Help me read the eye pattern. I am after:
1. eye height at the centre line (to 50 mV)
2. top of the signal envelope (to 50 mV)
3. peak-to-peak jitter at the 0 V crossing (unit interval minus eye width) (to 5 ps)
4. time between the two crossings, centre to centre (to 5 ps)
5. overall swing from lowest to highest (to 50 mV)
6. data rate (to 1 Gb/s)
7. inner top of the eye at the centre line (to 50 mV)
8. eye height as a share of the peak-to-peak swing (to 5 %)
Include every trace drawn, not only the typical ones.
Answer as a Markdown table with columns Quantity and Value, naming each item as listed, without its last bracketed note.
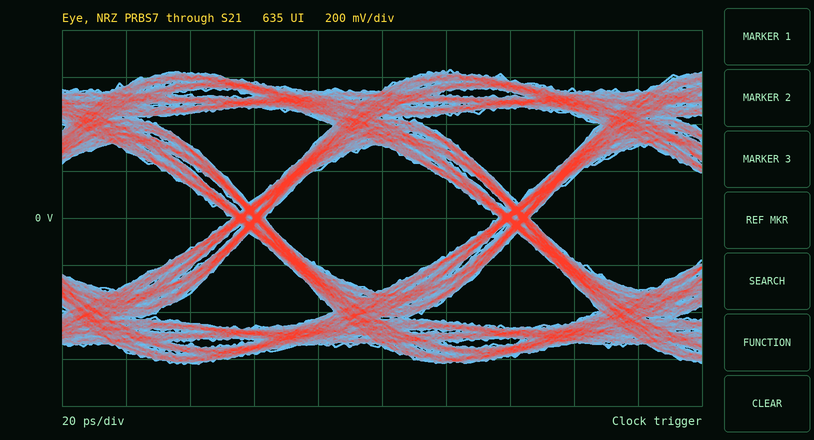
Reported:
| Quantity | Value |
|---|---|
| eye height at the centre line | 600 mV |
| top of the signal envelope | 650 mV |
| peak-to-peak jitter at the 0 V crossing (unit interval minus eye width) | 10 ps |
| time between the two crossings, centre to centre | 85 ps |
| overall swing from lowest to highest | 1.25 V |
| data rate | 12 Gb/s |
| inner top of the eye at the centre line | 300 mV |
| eye height as a share of the peak-to-peak swing | 50 % |
